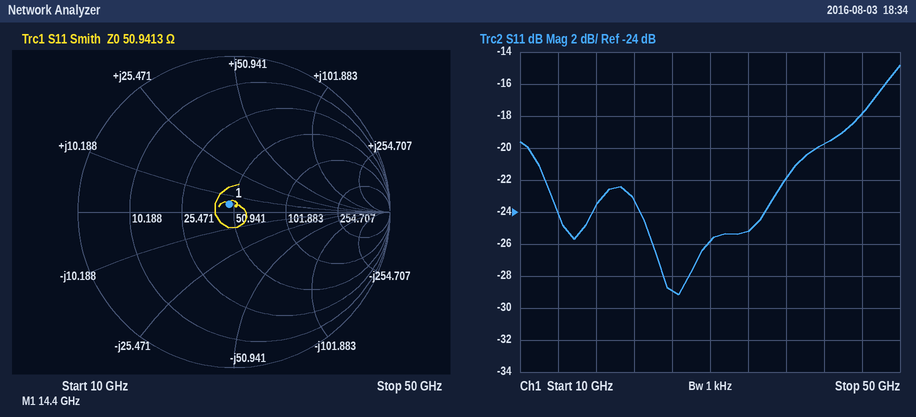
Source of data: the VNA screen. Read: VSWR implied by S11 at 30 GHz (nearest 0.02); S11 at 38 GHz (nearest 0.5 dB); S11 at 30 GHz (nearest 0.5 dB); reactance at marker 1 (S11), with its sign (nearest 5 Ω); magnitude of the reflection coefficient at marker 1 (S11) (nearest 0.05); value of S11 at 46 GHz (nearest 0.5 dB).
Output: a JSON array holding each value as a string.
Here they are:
["1.10", "-22.0 dB", "-26.0 dB", "+5 Ω", "0.05", "-18.0 dB"]
